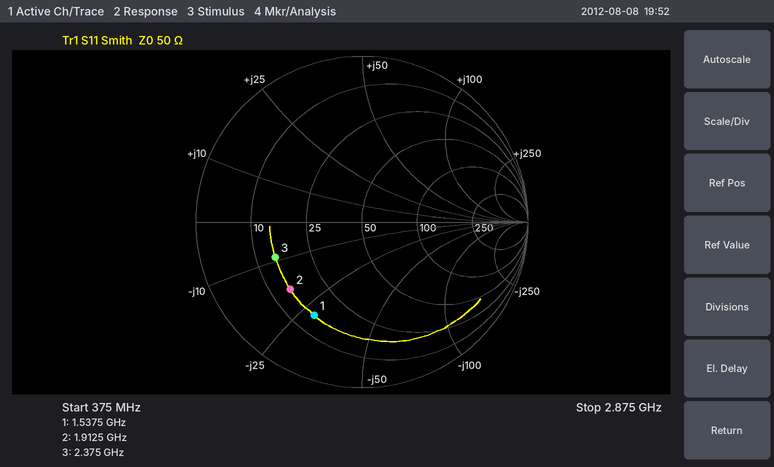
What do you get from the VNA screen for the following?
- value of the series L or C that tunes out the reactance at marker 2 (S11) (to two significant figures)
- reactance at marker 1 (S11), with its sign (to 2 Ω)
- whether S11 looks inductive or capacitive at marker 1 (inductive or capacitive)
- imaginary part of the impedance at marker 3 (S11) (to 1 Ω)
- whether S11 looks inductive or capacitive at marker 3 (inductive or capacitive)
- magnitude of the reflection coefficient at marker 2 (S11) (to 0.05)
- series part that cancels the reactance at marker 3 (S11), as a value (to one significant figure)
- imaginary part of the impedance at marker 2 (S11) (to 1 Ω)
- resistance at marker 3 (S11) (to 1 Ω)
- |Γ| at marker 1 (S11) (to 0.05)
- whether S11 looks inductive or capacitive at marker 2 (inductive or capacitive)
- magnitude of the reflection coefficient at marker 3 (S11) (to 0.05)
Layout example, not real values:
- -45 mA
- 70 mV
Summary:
- 1.5 nH
- -28 Ω
- capacitive
- -9 Ω
- capacitive
- 0.60
- 600 pH
- -18 Ω
- 14 Ω
- 0.65
- capacitive
- 0.55
